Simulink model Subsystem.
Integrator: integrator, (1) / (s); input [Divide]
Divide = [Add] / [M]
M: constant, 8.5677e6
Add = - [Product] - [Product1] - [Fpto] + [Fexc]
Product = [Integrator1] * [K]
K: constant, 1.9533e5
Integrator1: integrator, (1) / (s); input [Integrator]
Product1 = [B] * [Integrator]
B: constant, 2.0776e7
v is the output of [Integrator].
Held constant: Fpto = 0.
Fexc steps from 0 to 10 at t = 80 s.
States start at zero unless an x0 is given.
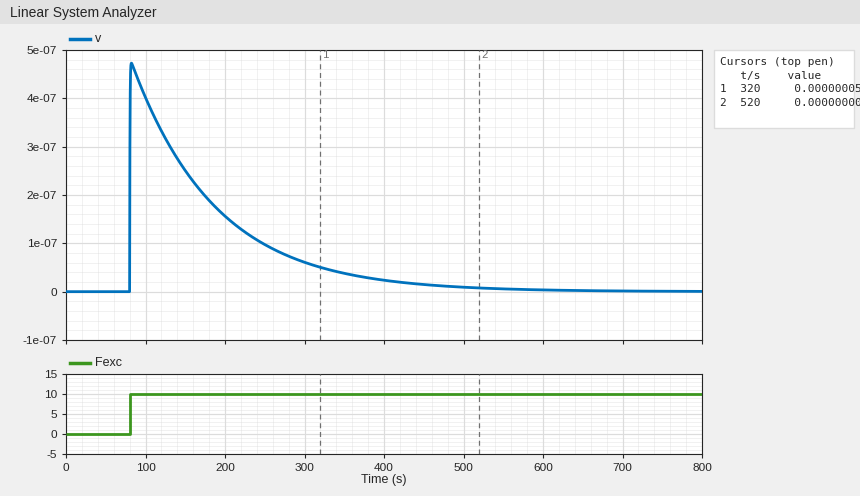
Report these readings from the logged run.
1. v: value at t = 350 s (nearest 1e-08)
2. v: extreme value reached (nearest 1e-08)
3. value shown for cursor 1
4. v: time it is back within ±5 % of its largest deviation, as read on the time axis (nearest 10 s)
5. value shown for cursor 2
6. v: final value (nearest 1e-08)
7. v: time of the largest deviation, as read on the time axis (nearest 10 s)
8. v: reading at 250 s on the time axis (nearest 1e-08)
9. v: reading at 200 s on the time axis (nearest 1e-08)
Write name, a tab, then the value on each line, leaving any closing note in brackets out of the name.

v: value at t = 350 s	0.00000004
v: extreme value reached	0.00000047
value shown for cursor 1	0.000000050
v: time it is back within ±5 % of its largest deviation, as read on the time axis	400 s
value shown for cursor 2	0.000000008
v: final value	0.00000000
v: time of the largest deviation, as read on the time axis	80 s
v: reading at 250 s on the time axis	0.00000010
v: reading at 200 s on the time axis	0.00000016
